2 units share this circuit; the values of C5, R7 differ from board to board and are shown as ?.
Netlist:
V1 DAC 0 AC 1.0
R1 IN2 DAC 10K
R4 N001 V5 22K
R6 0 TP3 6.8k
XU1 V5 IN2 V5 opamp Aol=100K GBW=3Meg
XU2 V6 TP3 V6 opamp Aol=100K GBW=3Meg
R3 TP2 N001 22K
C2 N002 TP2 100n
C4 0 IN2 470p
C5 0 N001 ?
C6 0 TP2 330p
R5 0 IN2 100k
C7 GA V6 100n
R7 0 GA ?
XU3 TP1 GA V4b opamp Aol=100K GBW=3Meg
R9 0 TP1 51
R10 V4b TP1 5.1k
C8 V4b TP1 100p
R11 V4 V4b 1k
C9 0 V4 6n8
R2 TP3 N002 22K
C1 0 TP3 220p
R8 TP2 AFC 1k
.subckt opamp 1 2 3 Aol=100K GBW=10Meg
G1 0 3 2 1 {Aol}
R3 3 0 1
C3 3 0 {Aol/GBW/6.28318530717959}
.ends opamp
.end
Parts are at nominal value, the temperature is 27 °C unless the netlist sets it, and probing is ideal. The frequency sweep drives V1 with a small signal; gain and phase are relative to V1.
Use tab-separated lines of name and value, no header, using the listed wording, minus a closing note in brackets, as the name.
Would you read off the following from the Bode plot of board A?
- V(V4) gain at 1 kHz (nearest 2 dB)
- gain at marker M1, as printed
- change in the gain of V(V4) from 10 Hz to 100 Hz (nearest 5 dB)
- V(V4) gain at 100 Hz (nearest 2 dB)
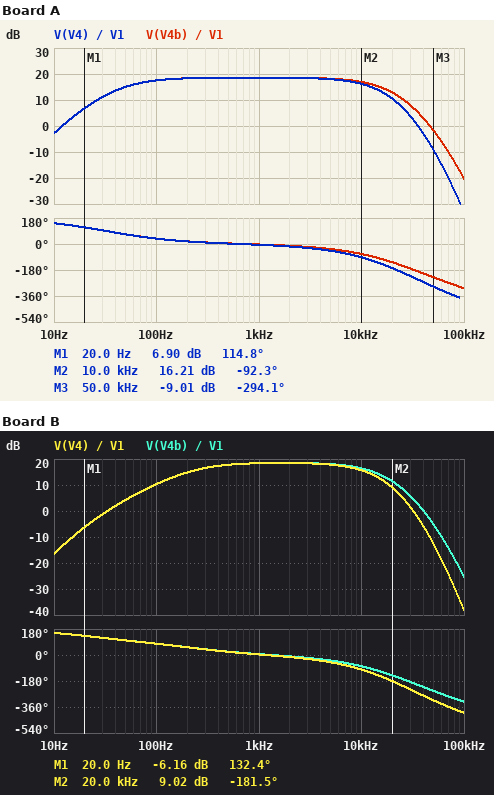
V(V4) gain at 1 kHz	18 dB
gain at marker M1, as printed	6.90 dB
change in the gain of V(V4) from 10 Hz to 100 Hz	20 dB
V(V4) gain at 100 Hz	18 dB
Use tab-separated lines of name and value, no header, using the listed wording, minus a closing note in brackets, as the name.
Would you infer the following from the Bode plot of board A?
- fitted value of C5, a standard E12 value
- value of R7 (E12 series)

fitted value of C5, a standard E12 value	180 pF
value of R7	33 kΩ
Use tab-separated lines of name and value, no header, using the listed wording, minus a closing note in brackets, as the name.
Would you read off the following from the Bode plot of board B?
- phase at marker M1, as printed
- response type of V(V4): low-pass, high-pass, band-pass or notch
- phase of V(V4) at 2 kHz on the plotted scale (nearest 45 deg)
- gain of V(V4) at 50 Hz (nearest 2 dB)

phase at marker M1, as printed	132.4 deg
response type of V(V4): low-pass, high-pass, band-pass or notch	band-pass
phase of V(V4) at 2 kHz on the plotted scale	0 deg
gain of V(V4) at 50 Hz	4 dB
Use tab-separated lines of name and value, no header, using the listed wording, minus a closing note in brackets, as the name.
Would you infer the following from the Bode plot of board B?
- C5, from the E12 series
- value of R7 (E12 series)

C5, from the E12 series	390 pF
value of R7	6.8 kΩ
